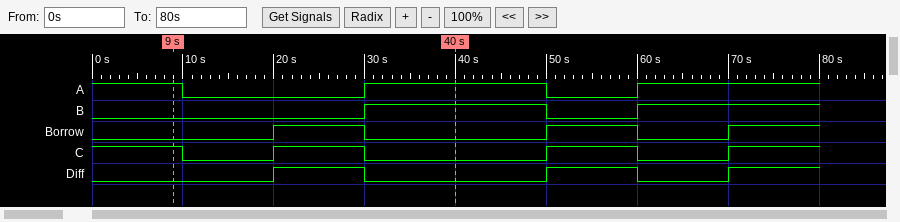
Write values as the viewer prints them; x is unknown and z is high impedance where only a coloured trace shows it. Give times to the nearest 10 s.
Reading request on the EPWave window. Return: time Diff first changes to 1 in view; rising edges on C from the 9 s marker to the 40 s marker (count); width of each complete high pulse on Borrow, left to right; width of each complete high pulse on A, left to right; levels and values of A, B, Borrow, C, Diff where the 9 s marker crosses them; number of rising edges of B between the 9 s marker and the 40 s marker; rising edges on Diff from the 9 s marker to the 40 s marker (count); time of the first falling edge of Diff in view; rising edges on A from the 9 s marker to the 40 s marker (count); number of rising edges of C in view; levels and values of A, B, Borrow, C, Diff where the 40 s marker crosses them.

20 s
1
10 s, 10 s
20 s
A=1, B=0, Borrow=0, C=1, Diff=0
1
1
30 s
1
3
A=1, B=1, Borrow=0, C=0, Diff=0
